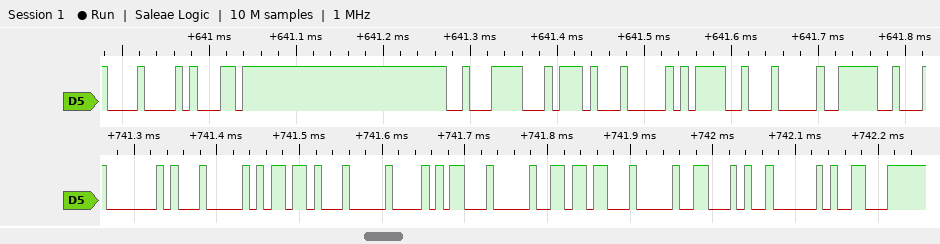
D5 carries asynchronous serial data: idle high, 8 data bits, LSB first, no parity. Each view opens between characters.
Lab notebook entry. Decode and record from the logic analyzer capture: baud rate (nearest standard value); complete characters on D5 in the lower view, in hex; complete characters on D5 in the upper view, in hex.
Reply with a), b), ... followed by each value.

a) 115200 baud
b) 40, 04, 6D, 04, A8, 04, B6, 04, 46, 02, 19
c) 08, B1, E2, 74, 04, 3D, 04, 3E
